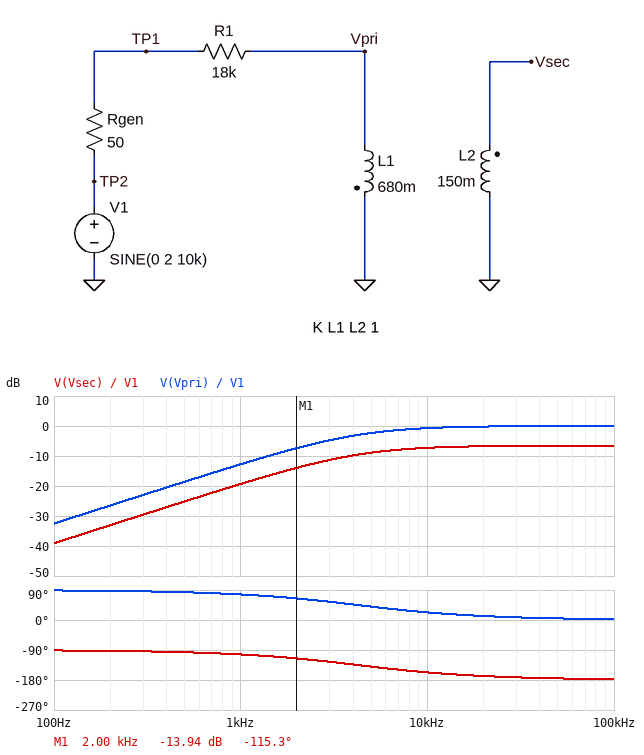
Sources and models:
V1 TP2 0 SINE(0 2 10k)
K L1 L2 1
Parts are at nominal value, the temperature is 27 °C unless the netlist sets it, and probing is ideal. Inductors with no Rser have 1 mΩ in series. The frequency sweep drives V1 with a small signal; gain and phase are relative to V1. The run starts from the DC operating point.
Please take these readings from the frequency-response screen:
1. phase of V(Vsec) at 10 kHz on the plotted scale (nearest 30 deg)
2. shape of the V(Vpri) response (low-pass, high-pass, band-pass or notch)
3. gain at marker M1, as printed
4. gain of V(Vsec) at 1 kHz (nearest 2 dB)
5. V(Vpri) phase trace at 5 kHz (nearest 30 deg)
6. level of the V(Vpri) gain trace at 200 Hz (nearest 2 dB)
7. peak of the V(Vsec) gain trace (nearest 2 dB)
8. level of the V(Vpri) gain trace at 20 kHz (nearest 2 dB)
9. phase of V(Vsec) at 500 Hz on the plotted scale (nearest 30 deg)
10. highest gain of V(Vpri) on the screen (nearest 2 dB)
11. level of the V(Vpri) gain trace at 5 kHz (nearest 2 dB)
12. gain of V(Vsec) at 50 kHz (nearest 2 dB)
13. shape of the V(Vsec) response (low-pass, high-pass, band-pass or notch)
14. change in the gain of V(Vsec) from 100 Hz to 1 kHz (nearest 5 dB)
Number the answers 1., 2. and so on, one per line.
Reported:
1. -150 deg
2. high-pass
3. -13.94 dB
4. -20 dB
5. 30 deg
6. -26 dB
7. -6 dB
8. 0 dB
9. -90 deg
10. 0 dB
11. -2 dB
12. -6 dB
13. high-pass
14. 20 dB
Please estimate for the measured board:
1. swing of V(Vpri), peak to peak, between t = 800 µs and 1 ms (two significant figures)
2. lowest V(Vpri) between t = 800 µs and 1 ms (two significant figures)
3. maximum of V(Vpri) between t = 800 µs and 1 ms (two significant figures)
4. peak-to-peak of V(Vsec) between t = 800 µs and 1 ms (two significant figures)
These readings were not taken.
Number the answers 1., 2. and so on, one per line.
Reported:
1. 3.7 V
2. -1.8 V
3. 1.8 V
4. 1.7 V
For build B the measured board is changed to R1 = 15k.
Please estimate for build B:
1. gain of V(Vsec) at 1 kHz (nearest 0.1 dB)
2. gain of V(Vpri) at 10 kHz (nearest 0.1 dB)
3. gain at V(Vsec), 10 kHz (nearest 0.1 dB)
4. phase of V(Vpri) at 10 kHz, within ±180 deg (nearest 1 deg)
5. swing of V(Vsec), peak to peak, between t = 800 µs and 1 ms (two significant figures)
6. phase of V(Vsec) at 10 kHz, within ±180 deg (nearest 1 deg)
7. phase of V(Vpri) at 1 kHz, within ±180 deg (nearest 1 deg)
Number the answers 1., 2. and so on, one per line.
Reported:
1. -17.8 dB
2. -0.5 dB
3. -7.1 dB
4. 19 deg
5. 1.8 V
6. -161 deg
7. 74 deg
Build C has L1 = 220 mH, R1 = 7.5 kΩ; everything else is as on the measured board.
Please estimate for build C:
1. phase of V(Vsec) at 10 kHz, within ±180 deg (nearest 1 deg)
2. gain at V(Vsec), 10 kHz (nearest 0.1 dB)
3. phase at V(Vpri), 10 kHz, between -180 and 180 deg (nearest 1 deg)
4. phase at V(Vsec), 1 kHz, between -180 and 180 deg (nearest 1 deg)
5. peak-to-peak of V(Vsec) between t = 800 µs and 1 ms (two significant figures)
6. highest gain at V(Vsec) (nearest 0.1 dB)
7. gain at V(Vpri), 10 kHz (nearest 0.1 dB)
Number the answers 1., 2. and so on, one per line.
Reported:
1. -151 deg
2. -2.8 dB
3. 29 deg
4. -100 deg
5. 2.9 V
6. -1.7 dB
7. -1.1 dB
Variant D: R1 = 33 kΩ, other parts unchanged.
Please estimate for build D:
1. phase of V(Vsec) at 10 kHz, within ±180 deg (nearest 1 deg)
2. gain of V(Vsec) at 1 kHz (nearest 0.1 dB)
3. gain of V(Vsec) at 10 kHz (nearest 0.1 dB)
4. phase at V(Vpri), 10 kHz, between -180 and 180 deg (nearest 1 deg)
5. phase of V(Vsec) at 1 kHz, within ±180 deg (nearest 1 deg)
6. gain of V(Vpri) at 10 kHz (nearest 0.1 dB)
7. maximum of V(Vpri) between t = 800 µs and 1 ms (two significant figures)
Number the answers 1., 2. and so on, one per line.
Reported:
1. -142 deg
2. -24.4 dB
3. -8.6 dB
4. 38 deg
5. -97 deg
6. -2.0 dB
7. 1.6 V
